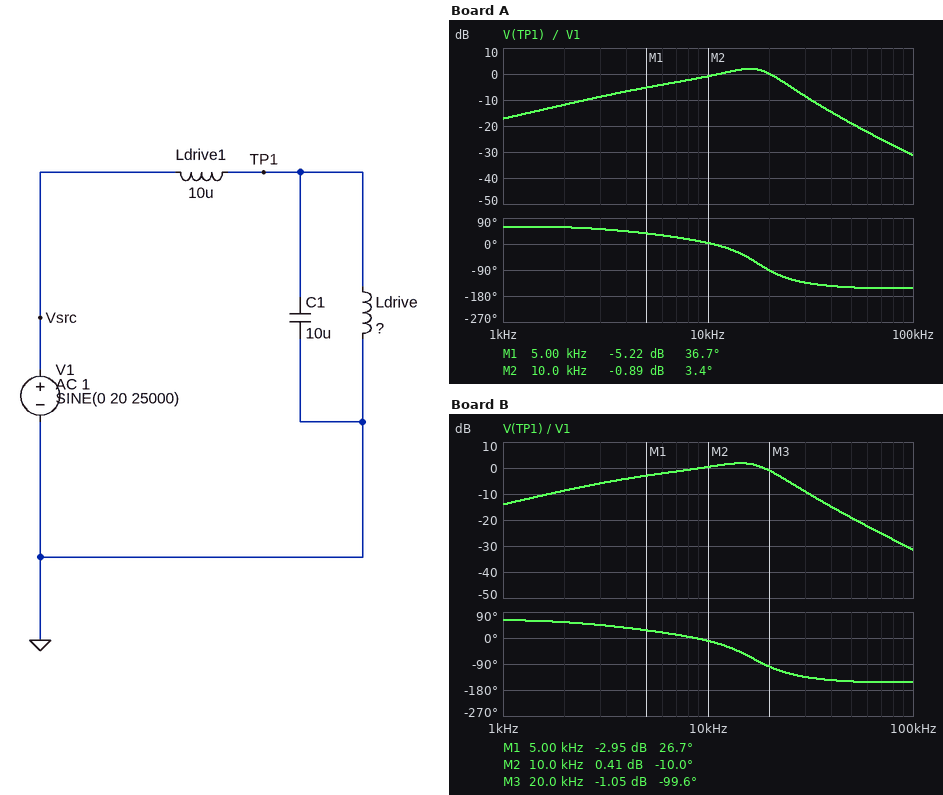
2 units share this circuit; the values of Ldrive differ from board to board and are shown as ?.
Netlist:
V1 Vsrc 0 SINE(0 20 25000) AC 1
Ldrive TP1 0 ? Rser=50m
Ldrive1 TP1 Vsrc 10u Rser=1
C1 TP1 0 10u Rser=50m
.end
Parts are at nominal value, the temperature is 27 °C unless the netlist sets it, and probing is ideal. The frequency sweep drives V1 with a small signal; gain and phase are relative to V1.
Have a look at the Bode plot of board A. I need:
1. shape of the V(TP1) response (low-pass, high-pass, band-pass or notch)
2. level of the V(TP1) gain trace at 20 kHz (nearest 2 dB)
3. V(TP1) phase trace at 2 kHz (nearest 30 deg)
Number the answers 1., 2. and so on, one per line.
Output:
1. band-pass
2. 0 dB
3. 60 deg
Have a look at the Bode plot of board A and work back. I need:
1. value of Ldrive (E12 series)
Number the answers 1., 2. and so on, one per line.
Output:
1. 22 µH
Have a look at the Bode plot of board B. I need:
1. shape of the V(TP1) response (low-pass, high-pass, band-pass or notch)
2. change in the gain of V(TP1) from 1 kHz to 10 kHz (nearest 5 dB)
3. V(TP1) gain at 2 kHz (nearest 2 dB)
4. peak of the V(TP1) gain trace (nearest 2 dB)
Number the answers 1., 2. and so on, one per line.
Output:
1. band-pass
2. 15 dB
3. -8 dB
4. 2 dB
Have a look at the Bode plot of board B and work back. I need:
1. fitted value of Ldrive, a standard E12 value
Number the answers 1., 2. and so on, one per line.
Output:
1. 33 µH
